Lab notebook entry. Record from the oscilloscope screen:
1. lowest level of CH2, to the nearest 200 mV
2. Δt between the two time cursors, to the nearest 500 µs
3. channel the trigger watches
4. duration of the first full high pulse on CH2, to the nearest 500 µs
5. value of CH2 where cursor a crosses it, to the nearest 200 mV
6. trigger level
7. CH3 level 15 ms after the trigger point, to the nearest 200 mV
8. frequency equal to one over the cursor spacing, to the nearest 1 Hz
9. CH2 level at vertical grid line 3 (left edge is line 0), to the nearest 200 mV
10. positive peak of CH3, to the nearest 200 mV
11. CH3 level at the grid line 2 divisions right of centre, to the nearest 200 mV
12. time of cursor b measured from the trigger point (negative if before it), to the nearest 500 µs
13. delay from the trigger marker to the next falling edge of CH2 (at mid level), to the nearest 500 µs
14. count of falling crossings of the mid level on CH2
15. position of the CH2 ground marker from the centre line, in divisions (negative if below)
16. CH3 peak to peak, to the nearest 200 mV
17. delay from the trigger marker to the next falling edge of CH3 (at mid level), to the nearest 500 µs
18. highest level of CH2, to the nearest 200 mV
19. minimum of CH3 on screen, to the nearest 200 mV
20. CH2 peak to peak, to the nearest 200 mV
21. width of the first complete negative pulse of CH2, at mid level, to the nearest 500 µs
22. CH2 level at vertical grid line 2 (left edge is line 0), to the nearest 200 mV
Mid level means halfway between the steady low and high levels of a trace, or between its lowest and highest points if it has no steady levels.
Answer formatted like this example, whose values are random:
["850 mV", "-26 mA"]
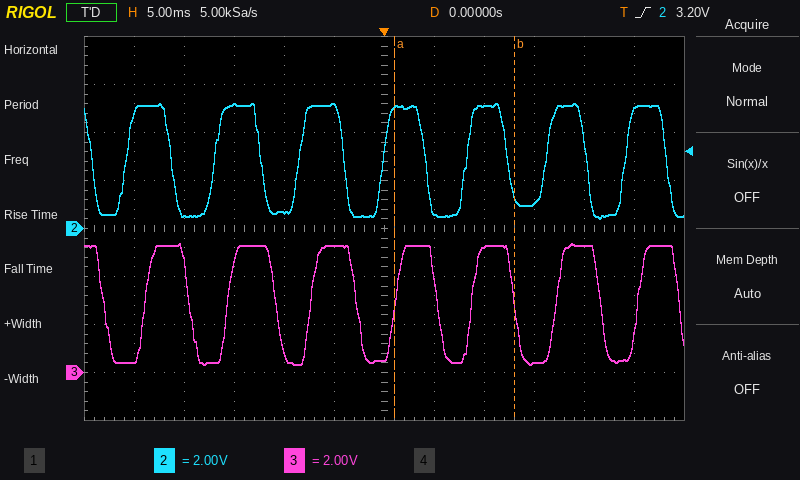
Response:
["400 mV", "12.0 ms", "CH2", "4.5 ms", "5.0 V", "3.20 V", "400 mV", "83 Hz", "5.2 V", "5.4 V", "5.2 V", "+13.0 ms", "4.0 ms", "8", "0.0 div", "5.0 V", "5.5 ms", "5.2 V", "400 mV", "4.8 V", "3.5 ms", "600 mV"]
